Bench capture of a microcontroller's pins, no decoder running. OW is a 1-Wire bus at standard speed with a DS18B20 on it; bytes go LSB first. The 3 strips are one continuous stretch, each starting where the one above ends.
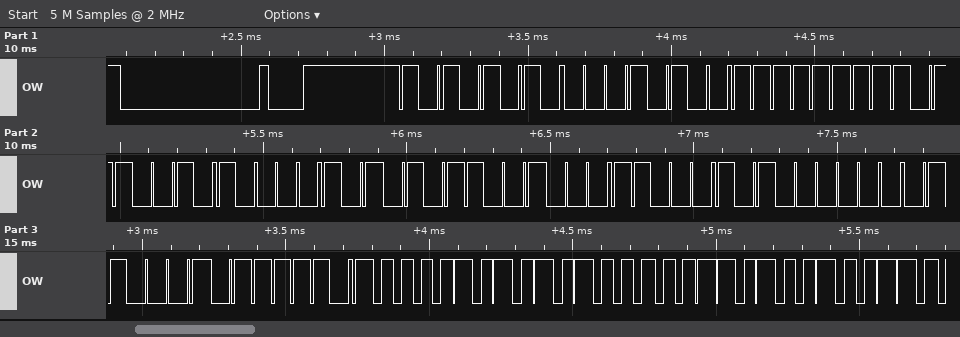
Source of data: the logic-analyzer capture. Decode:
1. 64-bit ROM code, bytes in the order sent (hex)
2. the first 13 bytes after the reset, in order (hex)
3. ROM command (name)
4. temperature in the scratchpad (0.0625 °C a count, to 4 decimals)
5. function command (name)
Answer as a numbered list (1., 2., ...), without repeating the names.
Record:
1. 28 FF 4D A1 9A 18 05 8C
2. 55 28 FF 4D A1 9A 18 05 8C BE 50 05 4B
3. Match ROM
4. 85.0000 °C
5. Read Scratchpad
